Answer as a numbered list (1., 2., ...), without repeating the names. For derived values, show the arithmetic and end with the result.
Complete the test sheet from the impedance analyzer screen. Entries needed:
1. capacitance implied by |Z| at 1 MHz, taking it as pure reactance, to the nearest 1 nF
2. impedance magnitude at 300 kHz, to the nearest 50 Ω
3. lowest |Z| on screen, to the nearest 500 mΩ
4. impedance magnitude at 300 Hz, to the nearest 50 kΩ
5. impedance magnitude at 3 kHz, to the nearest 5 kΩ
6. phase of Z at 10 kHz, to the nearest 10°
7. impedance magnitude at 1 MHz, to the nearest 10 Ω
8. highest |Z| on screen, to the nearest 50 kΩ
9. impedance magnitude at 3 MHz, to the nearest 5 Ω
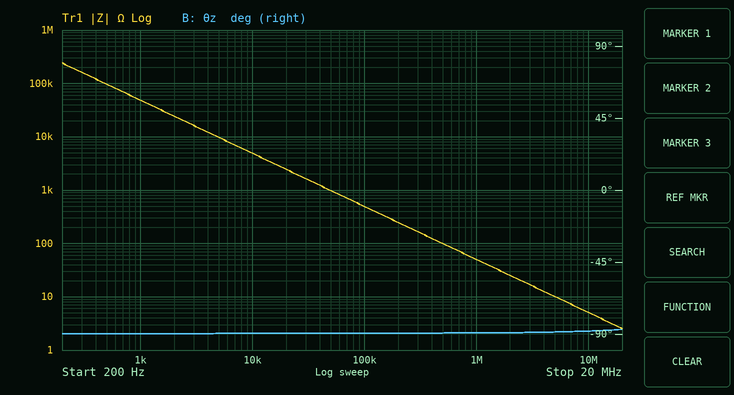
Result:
1. C = 1/(2π × 1 MHz × 50 Ω) ≈ 3 nF
2. 150 Ω
3. 2.5 Ω
4. 150 kΩ
5. 15 kΩ
6. -90°
7. 50 Ω
8. 250 kΩ
9. 15 Ω
